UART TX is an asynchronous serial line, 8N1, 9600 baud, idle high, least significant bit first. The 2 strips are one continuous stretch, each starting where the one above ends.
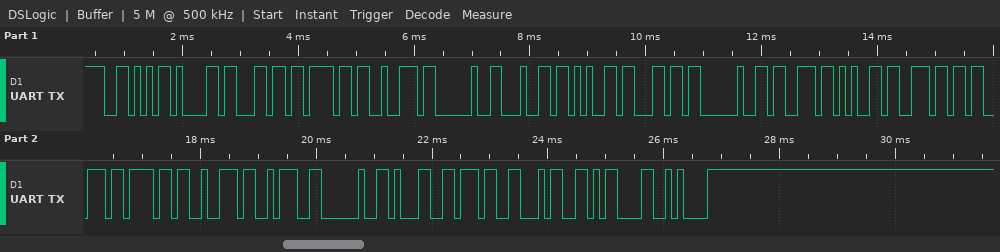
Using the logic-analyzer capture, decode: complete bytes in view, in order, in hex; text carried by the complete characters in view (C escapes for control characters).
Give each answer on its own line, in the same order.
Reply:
0x56 0x61 0x6C 0x6F 0x72 0x20 0x64 0x65 0x6C 0x20 0x73 0x65 0x6E 0x73 0x6F 0x72 0x3A 0x20 0x31 0x37 0x34 0x0D 0x0A
"Valor del sensor: 174\r\n"
